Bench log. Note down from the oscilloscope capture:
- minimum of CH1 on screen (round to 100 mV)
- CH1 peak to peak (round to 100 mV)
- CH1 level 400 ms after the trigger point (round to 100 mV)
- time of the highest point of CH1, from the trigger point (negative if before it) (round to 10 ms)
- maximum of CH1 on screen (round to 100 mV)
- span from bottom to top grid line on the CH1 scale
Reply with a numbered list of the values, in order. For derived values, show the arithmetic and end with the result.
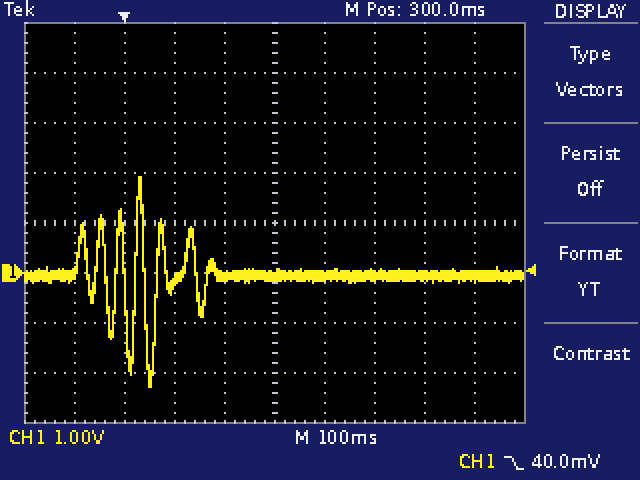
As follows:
1. -2.3 V
2. 1.9 V − (-2.3 V) = 4.2 V
3. -100 mV
4. +30 ms
5. 1.9 V
6. 8 V
